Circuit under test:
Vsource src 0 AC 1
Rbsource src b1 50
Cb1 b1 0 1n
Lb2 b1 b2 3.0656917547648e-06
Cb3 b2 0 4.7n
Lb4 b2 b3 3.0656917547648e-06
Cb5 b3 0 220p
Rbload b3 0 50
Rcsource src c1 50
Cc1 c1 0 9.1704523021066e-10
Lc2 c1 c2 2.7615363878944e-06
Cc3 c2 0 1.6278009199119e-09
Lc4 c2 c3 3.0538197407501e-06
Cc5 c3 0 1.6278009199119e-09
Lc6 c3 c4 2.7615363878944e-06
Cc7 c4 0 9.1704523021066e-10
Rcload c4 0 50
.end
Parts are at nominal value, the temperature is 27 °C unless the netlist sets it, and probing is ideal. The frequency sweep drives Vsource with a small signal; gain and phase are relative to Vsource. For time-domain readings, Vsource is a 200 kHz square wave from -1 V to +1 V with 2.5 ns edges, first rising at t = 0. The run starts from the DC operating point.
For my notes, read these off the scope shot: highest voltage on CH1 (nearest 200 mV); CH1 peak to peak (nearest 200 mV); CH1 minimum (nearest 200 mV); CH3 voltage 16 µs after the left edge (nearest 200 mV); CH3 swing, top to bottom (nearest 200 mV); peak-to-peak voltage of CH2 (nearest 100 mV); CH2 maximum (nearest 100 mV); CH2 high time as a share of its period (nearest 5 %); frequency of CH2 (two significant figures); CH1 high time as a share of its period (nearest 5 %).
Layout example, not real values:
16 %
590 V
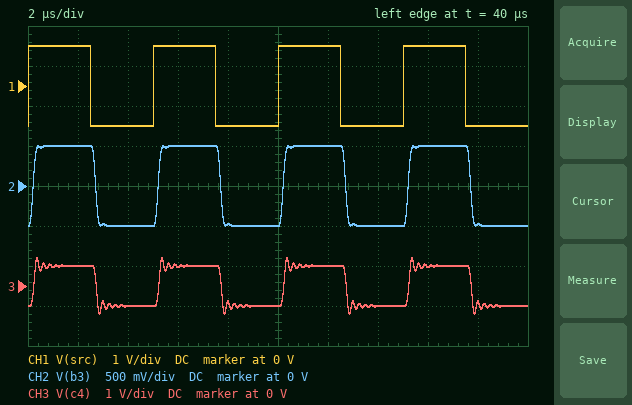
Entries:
1.0 V
2.0 V
-1.0 V
400 mV
1.4 V
1.0 V
500 mV
50 %
200 kHz
50 %
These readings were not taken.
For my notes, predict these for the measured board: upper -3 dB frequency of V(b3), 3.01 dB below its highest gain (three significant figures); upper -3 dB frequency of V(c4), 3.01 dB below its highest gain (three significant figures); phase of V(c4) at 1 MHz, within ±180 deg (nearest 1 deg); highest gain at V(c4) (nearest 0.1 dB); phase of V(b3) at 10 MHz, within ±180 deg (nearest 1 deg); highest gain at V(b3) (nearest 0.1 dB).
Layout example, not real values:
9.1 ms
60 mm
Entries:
1.83 MHz
4.38 MHz
-76 deg
-6.0 dB
-4 deg
-6.0 dB
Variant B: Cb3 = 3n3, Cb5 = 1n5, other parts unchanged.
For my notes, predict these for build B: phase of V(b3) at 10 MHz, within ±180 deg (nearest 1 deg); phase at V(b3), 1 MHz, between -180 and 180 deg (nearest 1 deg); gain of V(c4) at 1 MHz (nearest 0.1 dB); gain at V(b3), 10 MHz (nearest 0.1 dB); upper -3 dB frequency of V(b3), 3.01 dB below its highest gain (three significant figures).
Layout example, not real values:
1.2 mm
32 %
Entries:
-58 deg
-71 deg
-6.1 dB
-66.1 dB
3.11 MHz
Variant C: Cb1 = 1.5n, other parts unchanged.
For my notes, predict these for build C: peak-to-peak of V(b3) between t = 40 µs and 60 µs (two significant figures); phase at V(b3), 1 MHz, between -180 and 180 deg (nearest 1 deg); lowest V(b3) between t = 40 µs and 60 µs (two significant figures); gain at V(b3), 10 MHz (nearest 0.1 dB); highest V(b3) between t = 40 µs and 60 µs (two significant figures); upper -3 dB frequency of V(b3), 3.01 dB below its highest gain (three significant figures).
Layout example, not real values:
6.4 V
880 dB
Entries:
1.0 V
-76 deg
-510 mV
-60.4 dB
510 mV
2.21 MHz
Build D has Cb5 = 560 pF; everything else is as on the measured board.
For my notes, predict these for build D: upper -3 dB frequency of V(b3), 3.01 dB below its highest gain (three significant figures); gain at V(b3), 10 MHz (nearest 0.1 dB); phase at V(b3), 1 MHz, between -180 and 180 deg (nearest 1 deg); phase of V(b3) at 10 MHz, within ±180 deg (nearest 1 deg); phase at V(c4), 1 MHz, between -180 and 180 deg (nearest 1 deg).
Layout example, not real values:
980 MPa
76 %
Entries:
2.04 MHz
-61.3 dB
-75 deg
-37 deg
-76 deg
